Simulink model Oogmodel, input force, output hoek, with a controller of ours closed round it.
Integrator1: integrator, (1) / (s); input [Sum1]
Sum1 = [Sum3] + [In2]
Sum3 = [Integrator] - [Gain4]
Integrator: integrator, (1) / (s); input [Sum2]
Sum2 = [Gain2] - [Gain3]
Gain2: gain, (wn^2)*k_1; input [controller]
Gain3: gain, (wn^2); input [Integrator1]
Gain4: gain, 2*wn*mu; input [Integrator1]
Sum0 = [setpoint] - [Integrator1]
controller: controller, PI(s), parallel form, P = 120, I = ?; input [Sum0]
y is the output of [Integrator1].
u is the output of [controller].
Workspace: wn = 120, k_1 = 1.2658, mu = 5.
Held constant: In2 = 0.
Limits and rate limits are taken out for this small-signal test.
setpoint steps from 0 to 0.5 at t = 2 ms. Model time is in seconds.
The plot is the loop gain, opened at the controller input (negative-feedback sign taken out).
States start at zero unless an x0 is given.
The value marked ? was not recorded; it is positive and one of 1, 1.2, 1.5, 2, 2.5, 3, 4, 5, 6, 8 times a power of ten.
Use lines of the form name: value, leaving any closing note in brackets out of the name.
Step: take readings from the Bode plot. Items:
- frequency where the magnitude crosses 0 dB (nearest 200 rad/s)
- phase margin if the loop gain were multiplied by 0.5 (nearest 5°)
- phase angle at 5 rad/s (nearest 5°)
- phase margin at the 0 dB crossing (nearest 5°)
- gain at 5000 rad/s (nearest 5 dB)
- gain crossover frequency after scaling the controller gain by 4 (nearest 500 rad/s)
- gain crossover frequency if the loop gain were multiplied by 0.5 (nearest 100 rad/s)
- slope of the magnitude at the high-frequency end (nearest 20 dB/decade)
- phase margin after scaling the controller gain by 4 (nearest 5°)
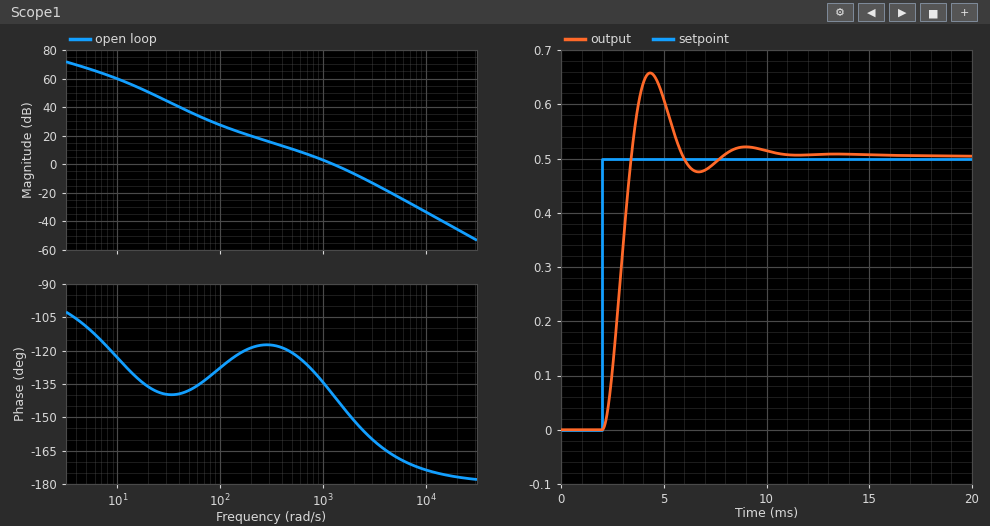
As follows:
frequency where the magnitude crosses 0 dB: 1200 rad/s
phase margin if the loop gain were multiplied by 0.5: 50°
phase angle at 5 rad/s: -110°
phase margin at the 0 dB crossing: 40°
gain at 5000 rad/s: -20 dB
gain crossover frequency after scaling the controller gain by 4: 3000 rad/s
gain crossover frequency if the loop gain were multiplied by 0.5: 800 rad/s
slope of the magnitude at the high-frequency end: -40 dB/decade
phase margin after scaling the controller gain by 4: 20°
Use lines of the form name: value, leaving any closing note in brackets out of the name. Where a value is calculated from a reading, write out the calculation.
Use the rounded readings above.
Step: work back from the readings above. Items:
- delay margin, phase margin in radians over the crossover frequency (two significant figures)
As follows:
delay margin, phase margin in radians over the crossover frequency: 40 × π / 180 / 1200 = 0.00058 s
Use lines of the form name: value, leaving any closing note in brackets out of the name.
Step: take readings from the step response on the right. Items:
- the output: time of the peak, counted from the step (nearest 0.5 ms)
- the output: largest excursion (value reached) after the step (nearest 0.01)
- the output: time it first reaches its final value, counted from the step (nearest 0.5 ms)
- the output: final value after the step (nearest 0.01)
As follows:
the output: time of the peak, counted from the step: 2.5 ms
the output: largest excursion (value reached) after the step: 0.66
the output: time it first reaches its final value, counted from the step: 1.5 ms
the output: final value after the step: 0.50
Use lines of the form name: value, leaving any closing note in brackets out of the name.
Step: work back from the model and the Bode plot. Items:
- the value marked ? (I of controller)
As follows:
the value marked ?: 10000
